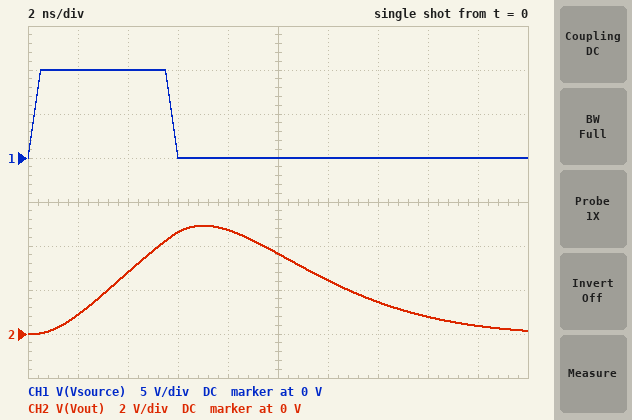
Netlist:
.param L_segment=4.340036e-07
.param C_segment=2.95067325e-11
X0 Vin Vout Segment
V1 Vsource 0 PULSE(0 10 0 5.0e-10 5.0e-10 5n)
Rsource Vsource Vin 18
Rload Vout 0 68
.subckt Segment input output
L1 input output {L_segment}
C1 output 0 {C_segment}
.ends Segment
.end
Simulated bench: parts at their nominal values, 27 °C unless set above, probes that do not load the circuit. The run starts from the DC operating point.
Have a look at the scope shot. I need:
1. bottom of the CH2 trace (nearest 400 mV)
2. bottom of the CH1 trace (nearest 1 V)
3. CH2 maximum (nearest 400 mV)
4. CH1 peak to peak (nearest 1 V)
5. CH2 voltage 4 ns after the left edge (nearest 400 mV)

0 V
0 V
4.8 V
10 V
2.8 V
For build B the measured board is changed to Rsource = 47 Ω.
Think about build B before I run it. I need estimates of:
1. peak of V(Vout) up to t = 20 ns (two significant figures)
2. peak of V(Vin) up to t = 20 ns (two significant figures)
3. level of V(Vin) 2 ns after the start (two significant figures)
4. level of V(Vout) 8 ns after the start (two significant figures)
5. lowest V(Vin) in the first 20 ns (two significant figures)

4.2 V
9.7 V
8.3 V
3.8 V
-3.4 V
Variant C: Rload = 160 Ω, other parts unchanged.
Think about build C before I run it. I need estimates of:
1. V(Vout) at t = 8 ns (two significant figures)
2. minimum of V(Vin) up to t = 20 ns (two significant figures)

7.6 V
-1.4 V
